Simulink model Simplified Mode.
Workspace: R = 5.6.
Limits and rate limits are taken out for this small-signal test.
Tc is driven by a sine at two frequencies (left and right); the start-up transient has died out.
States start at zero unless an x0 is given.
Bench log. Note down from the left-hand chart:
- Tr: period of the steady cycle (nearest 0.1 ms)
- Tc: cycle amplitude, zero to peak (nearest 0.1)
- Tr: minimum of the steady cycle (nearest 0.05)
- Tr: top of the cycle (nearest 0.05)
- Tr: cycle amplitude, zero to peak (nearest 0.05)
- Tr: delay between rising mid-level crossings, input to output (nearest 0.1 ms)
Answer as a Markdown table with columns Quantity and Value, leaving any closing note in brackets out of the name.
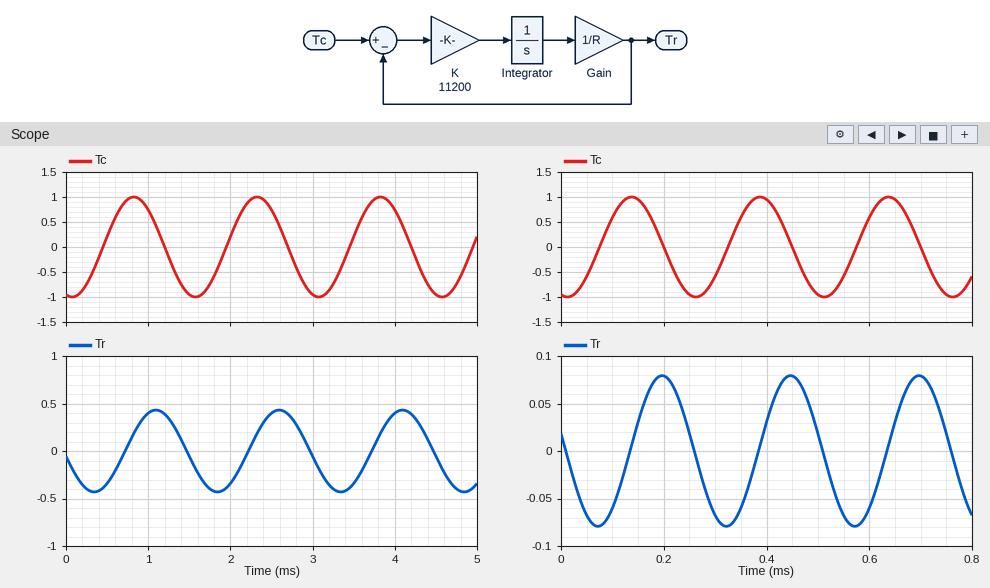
| Quantity | Value |
|---|---|
| Tr: period of the steady cycle | 1.5 ms |
| Tc: cycle amplitude, zero to peak | 1.0 |
| Tr: minimum of the steady cycle | -0.45 |
| Tr: top of the cycle | 0.45 |
| Tr: cycle amplitude, zero to peak | 0.45 |
| Tr: delay between rising mid-level crossings, input to output | 0.3 ms |
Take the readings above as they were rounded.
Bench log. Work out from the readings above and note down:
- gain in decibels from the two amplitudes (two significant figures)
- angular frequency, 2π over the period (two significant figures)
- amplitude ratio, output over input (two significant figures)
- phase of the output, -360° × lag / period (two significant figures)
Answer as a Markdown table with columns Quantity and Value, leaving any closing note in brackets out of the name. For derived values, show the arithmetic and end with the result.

| Quantity | Value |
|---|---|
| gain in decibels from the two amplitudes | 20 log10(0.45 / 1) = -6.9 dB |
| angular frequency, 2π over the period | 2π / 1.5 = 4.2 rad/ms |
| amplitude ratio, output over input | 0.45 / 1 = 0.45 |
| phase of the output, -360° × lag / period | -360 × 0.3 / 1.5 = -72° |
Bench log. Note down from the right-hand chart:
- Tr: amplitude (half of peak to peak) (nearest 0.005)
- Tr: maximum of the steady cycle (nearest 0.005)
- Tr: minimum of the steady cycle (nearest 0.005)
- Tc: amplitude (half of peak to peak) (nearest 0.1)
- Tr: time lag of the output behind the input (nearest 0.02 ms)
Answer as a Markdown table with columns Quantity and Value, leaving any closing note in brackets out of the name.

| Quantity | Value |
|---|---|
| Tr: amplitude (half of peak to peak) | 0.080 |
| Tr: maximum of the steady cycle | 0.080 |
| Tr: minimum of the steady cycle | -0.080 |
| Tc: amplitude (half of peak to peak) | 1.0 |
| Tr: time lag of the output behind the input | 0.06 ms |
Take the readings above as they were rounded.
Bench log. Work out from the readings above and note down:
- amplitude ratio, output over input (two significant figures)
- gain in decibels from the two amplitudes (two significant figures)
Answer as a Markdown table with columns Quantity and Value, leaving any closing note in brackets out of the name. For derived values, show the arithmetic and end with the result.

| Quantity | Value |
|---|---|
| amplitude ratio, output over input | 0.08 / 1 = 0.080 |
| gain in decibels from the two amplitudes | 20 log10(0.08 / 1) = -22 dB |
